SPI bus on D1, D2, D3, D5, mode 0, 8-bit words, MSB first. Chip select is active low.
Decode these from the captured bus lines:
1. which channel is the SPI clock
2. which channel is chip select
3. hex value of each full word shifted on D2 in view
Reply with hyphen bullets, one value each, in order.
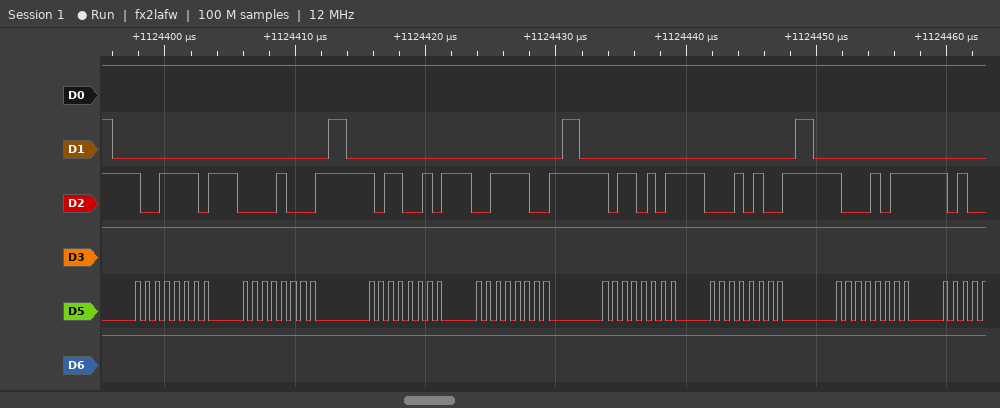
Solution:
- D5
- D1
- 9E, 08, B2, 3C, B5, 14, 8B
